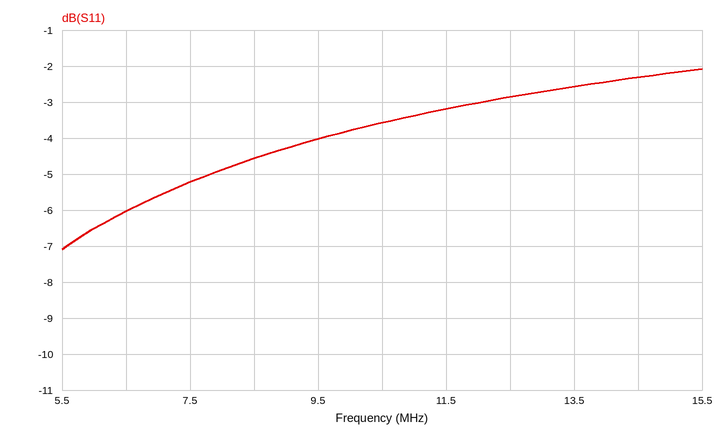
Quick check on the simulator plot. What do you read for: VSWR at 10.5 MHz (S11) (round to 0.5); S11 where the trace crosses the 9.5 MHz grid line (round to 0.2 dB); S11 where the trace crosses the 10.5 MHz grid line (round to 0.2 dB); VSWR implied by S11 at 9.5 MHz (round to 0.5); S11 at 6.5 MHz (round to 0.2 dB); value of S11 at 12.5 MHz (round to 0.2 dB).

5.0
-4.0 dB
-3.6 dB
4.5
-6.0 dB
-2.8 dB
